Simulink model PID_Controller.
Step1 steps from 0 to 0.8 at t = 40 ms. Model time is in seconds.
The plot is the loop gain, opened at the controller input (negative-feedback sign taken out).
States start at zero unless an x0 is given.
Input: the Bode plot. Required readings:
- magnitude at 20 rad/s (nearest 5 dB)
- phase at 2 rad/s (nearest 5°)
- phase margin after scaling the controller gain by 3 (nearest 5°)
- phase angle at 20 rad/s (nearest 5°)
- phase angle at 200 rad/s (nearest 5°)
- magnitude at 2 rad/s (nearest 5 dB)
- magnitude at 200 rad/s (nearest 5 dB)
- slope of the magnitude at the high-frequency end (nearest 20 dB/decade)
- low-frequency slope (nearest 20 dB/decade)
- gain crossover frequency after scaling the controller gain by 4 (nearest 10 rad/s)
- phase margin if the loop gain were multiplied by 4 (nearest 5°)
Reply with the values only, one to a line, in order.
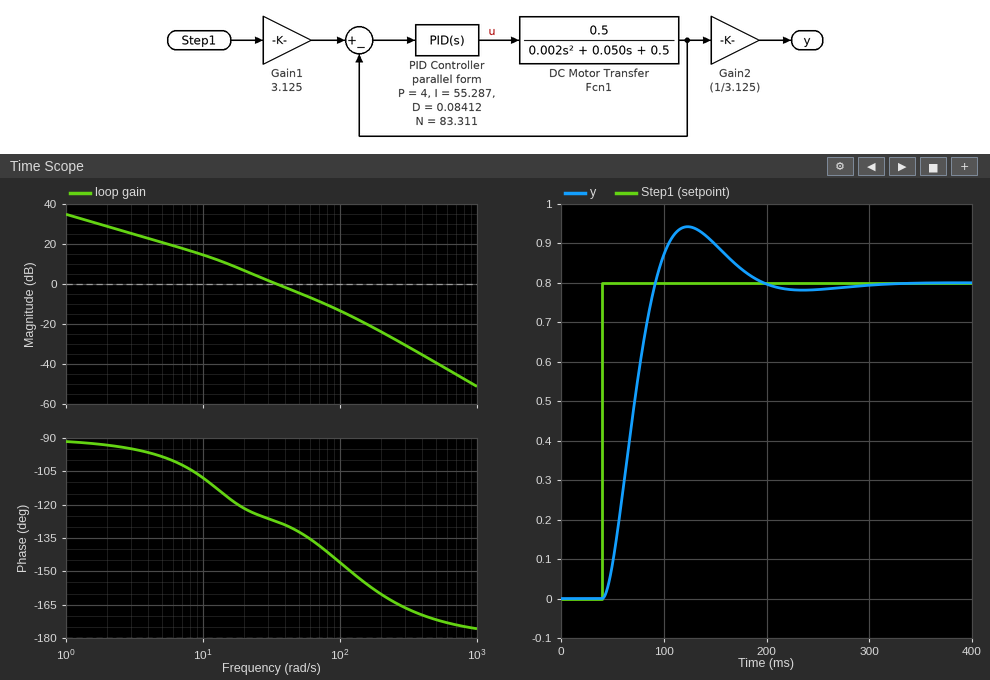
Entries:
5 dB
-95°
40°
-120°
-160°
30 dB
-25 dB
-40 dB/decade
-20 dB/decade
90 rad/s
35°
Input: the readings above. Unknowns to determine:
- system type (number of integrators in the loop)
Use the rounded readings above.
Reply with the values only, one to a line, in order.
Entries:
1
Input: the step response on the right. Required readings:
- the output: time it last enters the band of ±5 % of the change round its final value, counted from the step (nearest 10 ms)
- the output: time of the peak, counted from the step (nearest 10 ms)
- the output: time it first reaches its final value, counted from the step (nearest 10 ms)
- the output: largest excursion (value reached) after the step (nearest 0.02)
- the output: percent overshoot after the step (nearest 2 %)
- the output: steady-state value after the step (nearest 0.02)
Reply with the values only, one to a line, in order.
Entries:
130 ms
80 ms
50 ms
0.94
18 %
0.80
